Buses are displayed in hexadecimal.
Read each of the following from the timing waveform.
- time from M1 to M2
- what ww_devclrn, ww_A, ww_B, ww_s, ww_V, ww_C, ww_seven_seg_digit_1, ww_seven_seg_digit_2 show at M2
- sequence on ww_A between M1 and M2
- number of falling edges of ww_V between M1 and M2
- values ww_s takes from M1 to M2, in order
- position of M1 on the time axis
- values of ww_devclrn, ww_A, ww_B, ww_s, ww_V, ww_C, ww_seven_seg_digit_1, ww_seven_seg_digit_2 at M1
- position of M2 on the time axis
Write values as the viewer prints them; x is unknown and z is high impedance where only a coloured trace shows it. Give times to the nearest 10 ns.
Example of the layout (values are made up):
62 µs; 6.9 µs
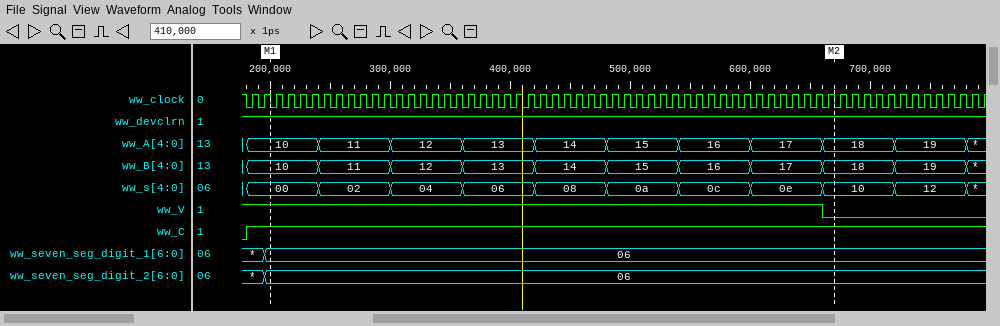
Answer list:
470 ns; ww_devclrn=1, ww_A=18, ww_B=18, ww_s=10, ww_V=0, ww_C=1, ww_seven_seg_digit_1=06, ww_seven_seg_digit_2=06; 10, 11, 12, 13, 14, 15, 16, 17, 18; 1; 00, 02, 04, 06, 08, 0a, 0c, 0e, 10; 200 ns; ww_devclrn=1, ww_A=10, ww_B=10, ww_s=00, ww_V=1, ww_C=1, ww_seven_seg_digit_1=06, ww_seven_seg_digit_2=06; 670 ns
